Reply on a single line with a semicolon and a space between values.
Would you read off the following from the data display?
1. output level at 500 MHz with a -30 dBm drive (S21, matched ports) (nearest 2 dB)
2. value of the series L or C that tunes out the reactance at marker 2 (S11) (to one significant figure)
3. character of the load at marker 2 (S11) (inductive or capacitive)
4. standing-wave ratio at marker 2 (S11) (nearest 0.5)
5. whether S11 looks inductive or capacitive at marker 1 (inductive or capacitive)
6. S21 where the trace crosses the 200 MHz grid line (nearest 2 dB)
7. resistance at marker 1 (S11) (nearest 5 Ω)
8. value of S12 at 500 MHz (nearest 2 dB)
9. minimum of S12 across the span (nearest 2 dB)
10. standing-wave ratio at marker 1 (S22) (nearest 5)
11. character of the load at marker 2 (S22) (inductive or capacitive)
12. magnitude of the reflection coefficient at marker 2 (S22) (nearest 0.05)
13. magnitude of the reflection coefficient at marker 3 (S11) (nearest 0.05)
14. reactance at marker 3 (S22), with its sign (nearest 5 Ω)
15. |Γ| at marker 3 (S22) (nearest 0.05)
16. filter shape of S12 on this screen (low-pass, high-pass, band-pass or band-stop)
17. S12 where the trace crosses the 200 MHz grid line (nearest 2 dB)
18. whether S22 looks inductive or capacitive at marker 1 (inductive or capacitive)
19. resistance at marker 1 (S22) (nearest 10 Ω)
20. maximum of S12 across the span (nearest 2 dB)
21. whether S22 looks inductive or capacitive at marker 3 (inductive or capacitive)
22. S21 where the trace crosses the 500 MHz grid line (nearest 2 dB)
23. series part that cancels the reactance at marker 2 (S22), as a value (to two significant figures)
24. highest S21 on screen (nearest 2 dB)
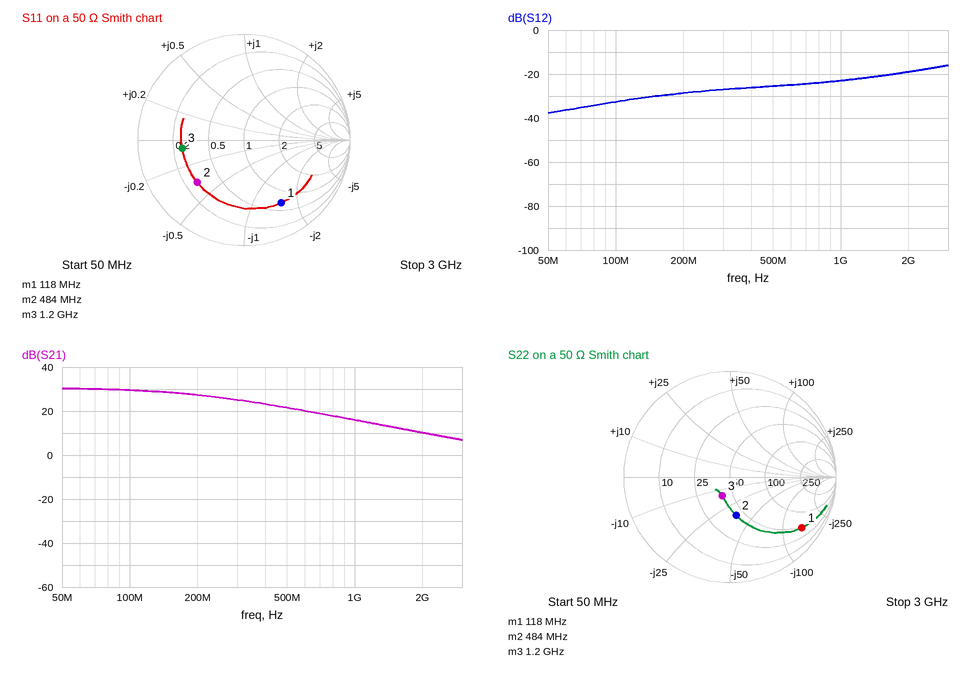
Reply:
-8 dBm; 6 nH; capacitive; 4.0; capacitive; 28 dB; 35 Ω; -26 dB; -38 dB; 10; capacitive; 0.35; 0.60; -15 Ω; 0.20; high-pass; -28 dB; capacitive; 50 Ω; -16 dB; capacitive; 22 dB; 12 nH; 30 dB
